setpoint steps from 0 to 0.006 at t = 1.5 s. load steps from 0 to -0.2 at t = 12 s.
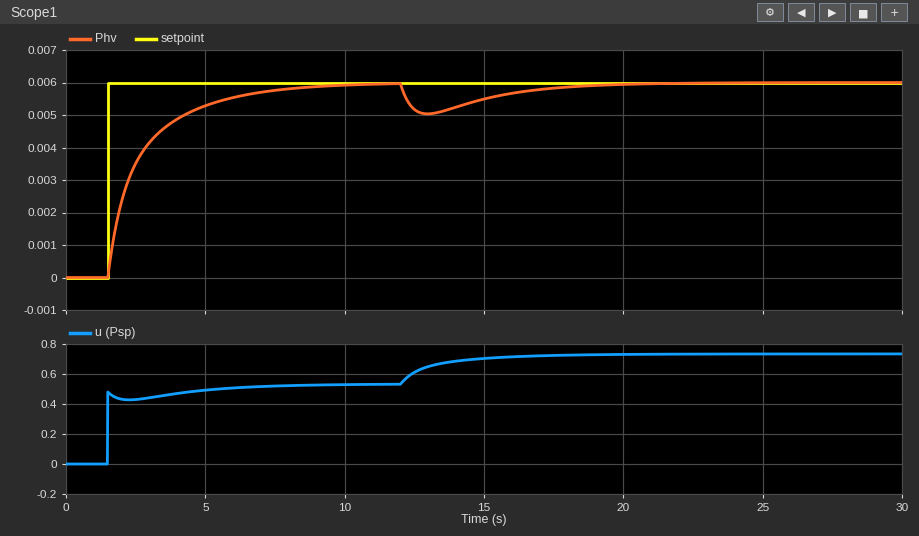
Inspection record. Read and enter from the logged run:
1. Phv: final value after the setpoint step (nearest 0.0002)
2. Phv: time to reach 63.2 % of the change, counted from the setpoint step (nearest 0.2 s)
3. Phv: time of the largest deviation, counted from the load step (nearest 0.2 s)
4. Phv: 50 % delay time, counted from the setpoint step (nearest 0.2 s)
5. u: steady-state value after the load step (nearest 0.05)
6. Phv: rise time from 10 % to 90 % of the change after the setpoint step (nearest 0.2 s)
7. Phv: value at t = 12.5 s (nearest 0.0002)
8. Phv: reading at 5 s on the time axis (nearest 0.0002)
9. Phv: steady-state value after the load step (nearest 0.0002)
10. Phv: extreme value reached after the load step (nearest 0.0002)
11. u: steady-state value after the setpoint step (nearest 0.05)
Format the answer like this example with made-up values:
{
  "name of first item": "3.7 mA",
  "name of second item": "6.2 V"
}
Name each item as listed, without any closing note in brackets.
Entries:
{
  "Phv: final value after the setpoint step": "0.0060",
  "Phv: time to reach 63.2 % of the change, counted from the setpoint step": "1.2 s",
  "Phv: time of the largest deviation, counted from the load step": "1.0 s",
  "Phv: 50 % delay time, counted from the setpoint step": "0.8 s",
  "u: steady-state value after the load step": "0.75",
  "Phv: rise time from 10 % to 90 % of the change after the setpoint step": "3.8 s",
  "Phv: value at t = 12.5 s": "0.0052",
  "Phv: reading at 5 s on the time axis": "0.0052",
  "Phv: steady-state value after the load step": "0.0060",
  "Phv: extreme value reached after the load step": "0.0050",
  "u: steady-state value after the setpoint step": "0.55"
}
